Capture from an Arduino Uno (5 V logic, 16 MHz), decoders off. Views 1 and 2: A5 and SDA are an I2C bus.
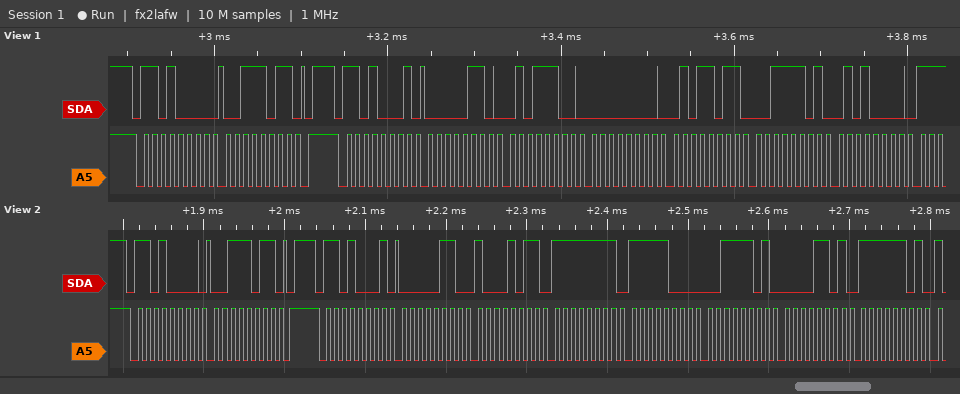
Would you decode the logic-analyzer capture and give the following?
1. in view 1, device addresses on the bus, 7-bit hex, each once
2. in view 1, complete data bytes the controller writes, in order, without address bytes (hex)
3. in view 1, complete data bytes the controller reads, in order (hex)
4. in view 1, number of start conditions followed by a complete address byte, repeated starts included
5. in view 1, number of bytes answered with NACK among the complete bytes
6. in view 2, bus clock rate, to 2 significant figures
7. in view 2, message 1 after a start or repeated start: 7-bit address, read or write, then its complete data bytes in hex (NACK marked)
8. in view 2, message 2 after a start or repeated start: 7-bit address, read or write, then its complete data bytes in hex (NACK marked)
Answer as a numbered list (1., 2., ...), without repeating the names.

1. 0x68
2. 3B
3. 06 5C 00 5B 3D 50
4. 2
5. 0
6. 100 kHz
7. 0x68 write: 3B
8. 0x68 read: 06 8B FF F8 3D 0D FD
